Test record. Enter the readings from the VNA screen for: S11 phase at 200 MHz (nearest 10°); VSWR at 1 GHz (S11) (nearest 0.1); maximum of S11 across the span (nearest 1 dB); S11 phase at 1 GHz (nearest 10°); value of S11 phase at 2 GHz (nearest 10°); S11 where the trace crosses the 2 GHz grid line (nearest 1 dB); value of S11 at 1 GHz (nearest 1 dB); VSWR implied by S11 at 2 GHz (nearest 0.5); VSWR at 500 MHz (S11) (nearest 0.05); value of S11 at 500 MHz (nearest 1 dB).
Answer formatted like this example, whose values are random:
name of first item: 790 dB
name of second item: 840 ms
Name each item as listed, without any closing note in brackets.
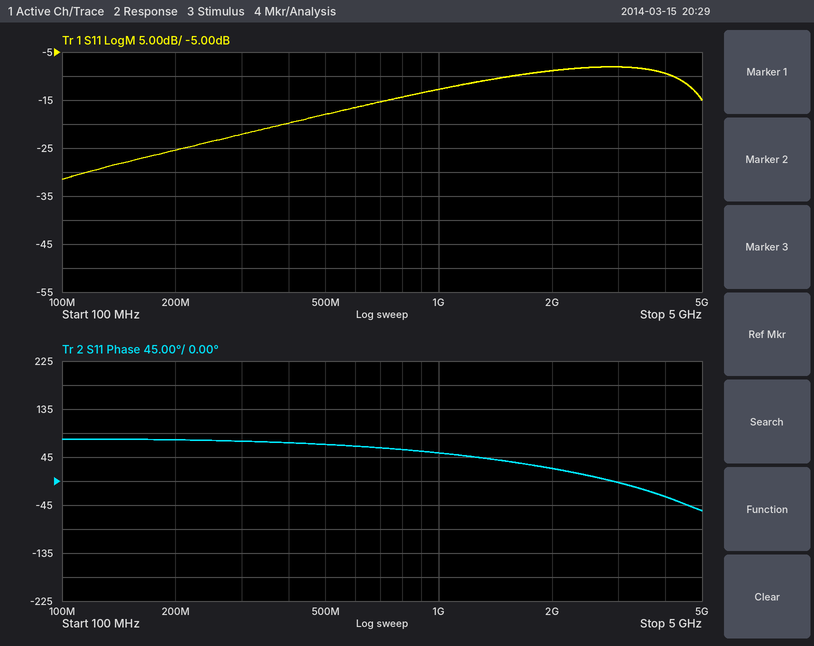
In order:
S11 phase at 200 MHz: 80°
VSWR at 1 GHz (S11): 1.6
maximum of S11 across the span: -8 dB
S11 phase at 1 GHz: 50°
value of S11 phase at 2 GHz: 20°
S11 where the trace crosses the 2 GHz grid line: -9 dB
value of S11 at 1 GHz: -13 dB
VSWR implied by S11 at 2 GHz: 2.0
VSWR at 500 MHz (S11): 1.30
value of S11 at 500 MHz: -18 dB
